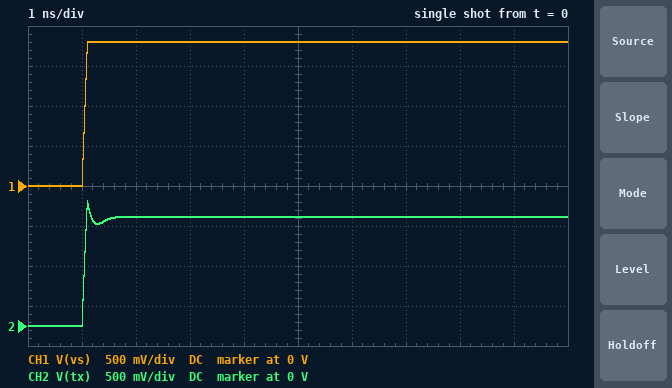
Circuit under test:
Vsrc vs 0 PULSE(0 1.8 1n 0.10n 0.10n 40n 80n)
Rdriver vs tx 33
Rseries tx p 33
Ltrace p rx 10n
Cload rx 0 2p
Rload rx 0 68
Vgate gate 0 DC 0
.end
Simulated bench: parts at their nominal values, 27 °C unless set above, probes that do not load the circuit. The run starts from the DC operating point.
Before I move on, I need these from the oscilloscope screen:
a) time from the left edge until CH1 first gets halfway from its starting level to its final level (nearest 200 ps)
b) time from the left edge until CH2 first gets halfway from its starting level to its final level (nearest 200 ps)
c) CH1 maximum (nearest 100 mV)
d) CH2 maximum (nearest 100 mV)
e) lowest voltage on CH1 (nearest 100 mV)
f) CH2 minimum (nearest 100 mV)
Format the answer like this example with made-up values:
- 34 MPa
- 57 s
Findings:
- 1.0 ns
- 1.0 ns
- 1.8 V
- 1.6 V
- 0 V
- 0 V
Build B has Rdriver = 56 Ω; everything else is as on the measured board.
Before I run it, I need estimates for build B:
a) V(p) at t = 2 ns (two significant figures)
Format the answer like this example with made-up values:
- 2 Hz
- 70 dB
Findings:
- 780 mV
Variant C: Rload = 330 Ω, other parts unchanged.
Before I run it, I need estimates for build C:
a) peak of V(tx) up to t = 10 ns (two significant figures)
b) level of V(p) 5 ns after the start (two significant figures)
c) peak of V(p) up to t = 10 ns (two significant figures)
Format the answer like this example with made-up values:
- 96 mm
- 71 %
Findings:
- 1.7 V
- 1.5 V
- 1.6 V
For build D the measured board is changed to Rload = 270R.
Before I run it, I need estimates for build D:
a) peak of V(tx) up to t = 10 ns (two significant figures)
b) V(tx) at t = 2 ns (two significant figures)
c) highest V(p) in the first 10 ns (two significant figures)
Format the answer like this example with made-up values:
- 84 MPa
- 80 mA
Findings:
- 1.7 V
- 1.6 V
- 1.5 V
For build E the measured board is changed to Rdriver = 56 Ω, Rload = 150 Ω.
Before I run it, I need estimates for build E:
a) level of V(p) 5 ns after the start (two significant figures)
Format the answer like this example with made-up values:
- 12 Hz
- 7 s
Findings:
- 1.1 V
